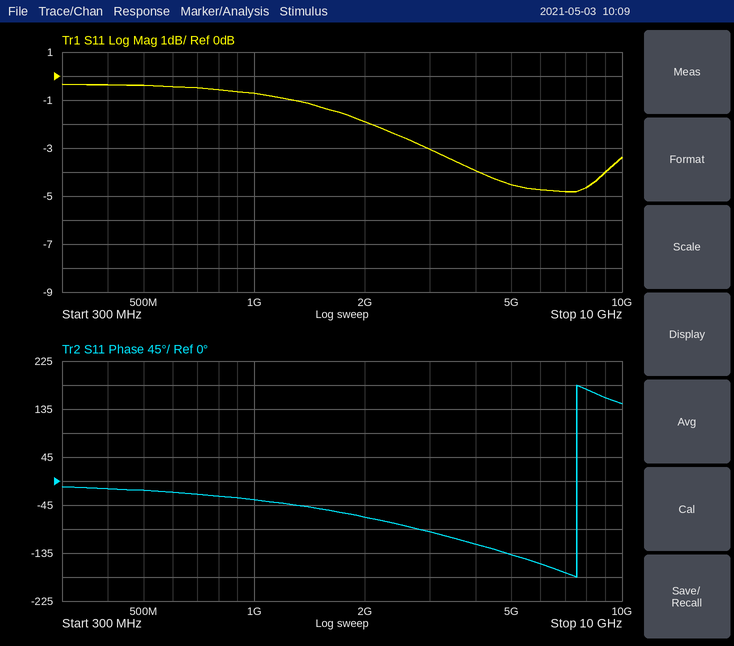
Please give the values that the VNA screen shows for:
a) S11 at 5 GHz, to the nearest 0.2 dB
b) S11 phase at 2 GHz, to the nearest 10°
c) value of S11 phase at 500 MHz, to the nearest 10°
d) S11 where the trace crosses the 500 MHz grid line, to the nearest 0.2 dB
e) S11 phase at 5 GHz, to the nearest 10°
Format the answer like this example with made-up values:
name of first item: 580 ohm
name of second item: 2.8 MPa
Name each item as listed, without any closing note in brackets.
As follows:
S11 at 5 GHz, to the nearest 0.2 dB: -4.6 dB
S11 phase at 2 GHz, to the nearest 10°: -70°
value of S11 phase at 500 MHz, to the nearest 10°: -20°
S11 where the trace crosses the 500 MHz grid line, to the nearest 0.2 dB: -0.4 dB
S11 phase at 5 GHz, to the nearest 10°: -140°
